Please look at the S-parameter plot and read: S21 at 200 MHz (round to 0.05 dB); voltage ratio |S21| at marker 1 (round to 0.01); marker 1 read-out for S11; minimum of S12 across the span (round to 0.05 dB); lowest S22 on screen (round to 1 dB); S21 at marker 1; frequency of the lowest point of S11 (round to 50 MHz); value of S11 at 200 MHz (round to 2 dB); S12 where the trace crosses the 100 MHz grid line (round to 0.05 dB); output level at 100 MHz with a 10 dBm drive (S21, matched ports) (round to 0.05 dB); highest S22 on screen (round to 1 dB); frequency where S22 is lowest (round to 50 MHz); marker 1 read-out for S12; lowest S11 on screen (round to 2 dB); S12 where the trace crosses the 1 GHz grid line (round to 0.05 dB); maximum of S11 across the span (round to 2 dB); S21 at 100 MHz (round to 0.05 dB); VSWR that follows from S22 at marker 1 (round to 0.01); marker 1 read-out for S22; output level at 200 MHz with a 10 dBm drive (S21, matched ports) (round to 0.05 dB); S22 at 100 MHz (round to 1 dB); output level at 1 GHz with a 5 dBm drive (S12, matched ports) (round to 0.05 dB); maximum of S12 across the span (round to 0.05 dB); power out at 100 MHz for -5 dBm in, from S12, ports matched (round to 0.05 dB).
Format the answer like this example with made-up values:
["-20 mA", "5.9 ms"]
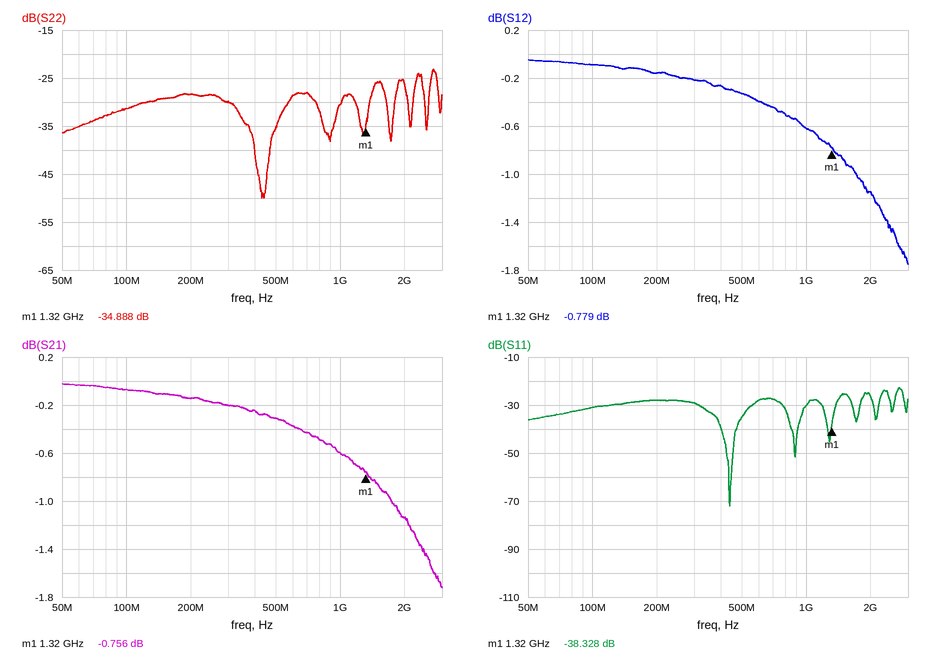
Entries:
["-0.15 dB", "0.92", "-38.328 dB", "-1.75 dB", "-50 dB", "-0.756 dB", "450 MHz", "-28 dB", "-0.10 dB", "9.95 dBm", "-23 dB", "450 MHz", "-0.779 dB", "-72 dB", "-0.60 dB", "-22 dB", "-0.05 dB", "1.04", "-34.888 dB", "9.85 dBm", "-31 dB", "4.40 dBm", "-0.05 dB", "-5.10 dBm"]
